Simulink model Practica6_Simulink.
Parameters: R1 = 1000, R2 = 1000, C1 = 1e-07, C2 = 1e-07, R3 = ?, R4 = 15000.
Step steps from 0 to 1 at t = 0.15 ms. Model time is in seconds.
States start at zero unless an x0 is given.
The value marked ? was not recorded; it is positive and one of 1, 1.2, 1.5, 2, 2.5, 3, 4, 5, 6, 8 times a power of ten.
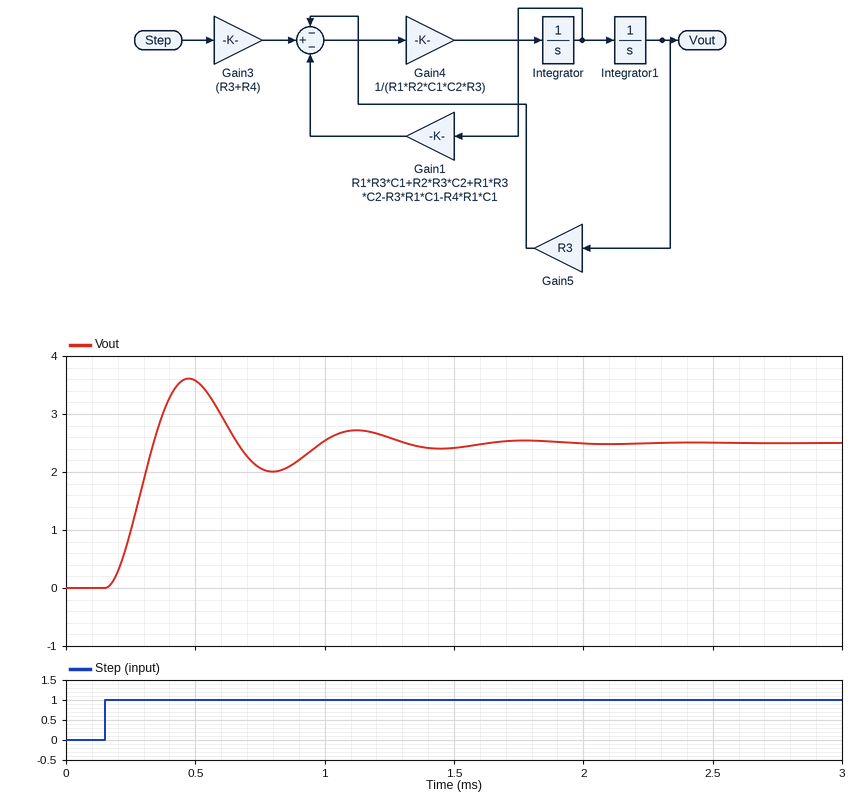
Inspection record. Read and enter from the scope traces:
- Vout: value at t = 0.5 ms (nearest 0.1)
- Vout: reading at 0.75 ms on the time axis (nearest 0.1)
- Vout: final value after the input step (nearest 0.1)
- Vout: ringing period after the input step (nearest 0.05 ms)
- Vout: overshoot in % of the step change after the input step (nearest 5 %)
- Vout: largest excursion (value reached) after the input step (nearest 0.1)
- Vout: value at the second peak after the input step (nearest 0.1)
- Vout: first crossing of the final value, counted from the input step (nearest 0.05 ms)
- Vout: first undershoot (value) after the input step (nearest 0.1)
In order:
3.6
2.1
2.5
0.65 ms
45 %
3.6
2.7
0.20 ms
2.0
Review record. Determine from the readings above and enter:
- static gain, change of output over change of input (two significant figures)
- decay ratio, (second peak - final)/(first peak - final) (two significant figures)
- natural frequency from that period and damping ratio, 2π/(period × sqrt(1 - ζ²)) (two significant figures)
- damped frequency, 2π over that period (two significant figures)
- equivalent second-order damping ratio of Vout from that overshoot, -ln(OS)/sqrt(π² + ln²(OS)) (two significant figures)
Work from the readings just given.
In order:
2.5
0.18
10.0 rad/ms
9.7 rad/ms
0.25
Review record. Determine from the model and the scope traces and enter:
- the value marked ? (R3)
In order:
10000
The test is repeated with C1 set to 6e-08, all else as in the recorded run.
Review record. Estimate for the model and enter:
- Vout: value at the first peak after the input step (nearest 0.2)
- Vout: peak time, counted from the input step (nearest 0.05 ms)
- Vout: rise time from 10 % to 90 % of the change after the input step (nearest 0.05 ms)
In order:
2.6
0.35 ms
0.15 ms
